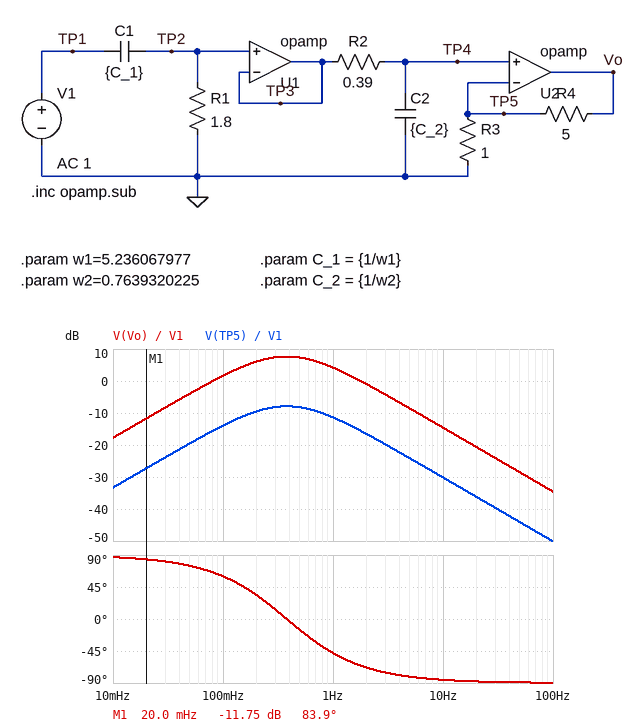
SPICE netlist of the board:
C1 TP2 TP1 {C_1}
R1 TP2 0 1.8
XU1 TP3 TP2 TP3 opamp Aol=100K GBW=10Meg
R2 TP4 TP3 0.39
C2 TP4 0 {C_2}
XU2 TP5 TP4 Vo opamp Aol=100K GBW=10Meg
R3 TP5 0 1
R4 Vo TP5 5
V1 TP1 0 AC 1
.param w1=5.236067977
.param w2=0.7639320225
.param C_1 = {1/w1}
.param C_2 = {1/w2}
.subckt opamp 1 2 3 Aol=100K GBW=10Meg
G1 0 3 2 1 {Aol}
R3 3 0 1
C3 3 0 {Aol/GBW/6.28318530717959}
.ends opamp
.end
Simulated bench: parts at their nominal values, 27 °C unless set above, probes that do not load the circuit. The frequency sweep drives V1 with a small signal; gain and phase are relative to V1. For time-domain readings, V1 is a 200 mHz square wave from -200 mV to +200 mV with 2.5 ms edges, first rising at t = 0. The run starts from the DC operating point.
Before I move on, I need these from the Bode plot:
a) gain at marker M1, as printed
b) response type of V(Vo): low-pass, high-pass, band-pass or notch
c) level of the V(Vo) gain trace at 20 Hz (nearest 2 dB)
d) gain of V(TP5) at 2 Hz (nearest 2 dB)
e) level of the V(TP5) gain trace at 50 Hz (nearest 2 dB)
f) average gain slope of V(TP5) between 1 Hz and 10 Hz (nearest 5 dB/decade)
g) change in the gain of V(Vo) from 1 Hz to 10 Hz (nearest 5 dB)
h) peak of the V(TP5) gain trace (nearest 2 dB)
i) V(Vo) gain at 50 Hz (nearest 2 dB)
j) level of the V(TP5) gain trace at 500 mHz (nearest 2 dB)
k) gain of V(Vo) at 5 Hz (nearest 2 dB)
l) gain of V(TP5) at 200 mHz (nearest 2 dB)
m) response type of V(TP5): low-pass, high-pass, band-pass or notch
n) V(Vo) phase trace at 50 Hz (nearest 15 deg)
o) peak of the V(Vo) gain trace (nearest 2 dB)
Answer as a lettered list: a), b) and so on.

a) -11.75 dB
b) band-pass
c) -20 dB
d) -16 dB
e) -44 dB
f) -20 dB/decade
g) -20 dB
h) -8 dB
i) -28 dB
j) -8 dB
k) -8 dB
l) -10 dB
m) band-pass
n) -90 deg
o) 8 dB
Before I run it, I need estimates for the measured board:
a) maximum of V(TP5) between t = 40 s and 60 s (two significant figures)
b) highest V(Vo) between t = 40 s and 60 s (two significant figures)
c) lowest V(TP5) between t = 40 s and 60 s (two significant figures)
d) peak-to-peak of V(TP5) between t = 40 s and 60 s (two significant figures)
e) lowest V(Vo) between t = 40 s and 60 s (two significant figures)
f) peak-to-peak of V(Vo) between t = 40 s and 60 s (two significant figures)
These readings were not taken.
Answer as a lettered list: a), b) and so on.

a) 120 mV
b) 700 mV
c) -120 mV
d) 230 mV
e) -700 mV
f) 1.4 V
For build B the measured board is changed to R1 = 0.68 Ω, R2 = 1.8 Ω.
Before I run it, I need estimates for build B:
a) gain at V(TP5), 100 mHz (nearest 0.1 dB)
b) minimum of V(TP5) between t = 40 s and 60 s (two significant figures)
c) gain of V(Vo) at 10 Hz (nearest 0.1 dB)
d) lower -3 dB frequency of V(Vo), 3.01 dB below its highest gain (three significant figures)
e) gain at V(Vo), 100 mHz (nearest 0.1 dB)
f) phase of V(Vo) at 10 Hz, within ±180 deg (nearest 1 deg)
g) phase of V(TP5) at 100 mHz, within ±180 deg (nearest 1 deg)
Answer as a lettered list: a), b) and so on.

a) -26.8 dB
b) -14 mV
c) -27.9 dB
d) 61.1 mHz
e) -11.3 dB
f) -83 deg
g) 29 deg
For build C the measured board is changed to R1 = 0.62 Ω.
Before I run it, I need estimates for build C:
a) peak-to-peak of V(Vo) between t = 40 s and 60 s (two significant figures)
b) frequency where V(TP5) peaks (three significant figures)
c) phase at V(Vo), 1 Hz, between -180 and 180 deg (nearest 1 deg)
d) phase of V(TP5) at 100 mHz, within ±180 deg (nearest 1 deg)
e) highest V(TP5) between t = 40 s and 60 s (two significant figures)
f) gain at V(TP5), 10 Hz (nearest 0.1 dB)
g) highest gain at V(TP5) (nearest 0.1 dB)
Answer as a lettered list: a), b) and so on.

a) 710 mV
b) 647 mHz
c) -19 deg
d) 68 deg
e) 59 mV
f) -30.2 dB
g) -14.5 dB
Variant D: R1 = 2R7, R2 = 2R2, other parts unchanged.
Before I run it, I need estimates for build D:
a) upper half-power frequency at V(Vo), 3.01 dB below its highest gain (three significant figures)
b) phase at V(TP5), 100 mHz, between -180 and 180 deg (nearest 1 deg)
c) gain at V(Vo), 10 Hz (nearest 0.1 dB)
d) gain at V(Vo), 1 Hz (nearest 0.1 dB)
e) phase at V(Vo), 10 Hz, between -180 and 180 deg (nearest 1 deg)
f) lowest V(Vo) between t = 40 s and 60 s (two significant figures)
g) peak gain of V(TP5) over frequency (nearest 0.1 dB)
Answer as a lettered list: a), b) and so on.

a) 406 mHz
b) 11 deg
c) -29.6 dB
d) -10.0 dB
e) -88 deg
f) -190 mV
g) -16.4 dB
